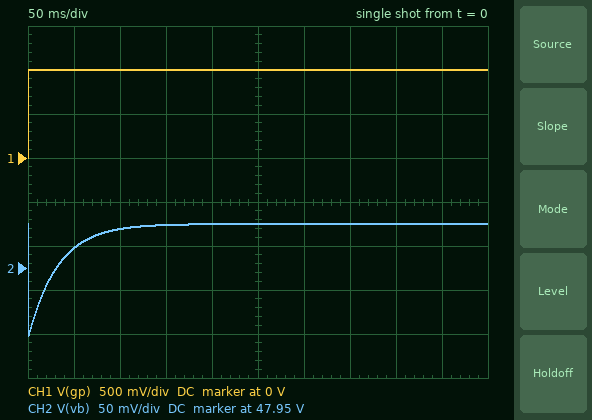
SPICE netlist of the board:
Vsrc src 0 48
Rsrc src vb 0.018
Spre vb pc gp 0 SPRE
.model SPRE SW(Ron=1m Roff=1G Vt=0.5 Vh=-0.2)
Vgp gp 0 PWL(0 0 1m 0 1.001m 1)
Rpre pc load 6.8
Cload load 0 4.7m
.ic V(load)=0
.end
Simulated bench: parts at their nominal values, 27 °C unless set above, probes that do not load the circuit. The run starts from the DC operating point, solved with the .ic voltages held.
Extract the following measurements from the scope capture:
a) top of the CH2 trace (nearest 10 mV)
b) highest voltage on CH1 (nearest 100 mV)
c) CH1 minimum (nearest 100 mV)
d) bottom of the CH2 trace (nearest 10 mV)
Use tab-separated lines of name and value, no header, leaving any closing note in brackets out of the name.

top of the CH2 trace	48.00 V
highest voltage on CH1	1.0 V
CH1 minimum	0 V
bottom of the CH2 trace	47.87 V
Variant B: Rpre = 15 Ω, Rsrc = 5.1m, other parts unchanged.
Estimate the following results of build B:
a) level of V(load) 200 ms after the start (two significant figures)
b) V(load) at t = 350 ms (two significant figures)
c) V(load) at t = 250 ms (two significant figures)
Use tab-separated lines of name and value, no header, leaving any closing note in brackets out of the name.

level of V(load) 200 ms after the start	45 V
V(load) at t = 350 ms	48 V
V(load) at t = 250 ms	47 V
